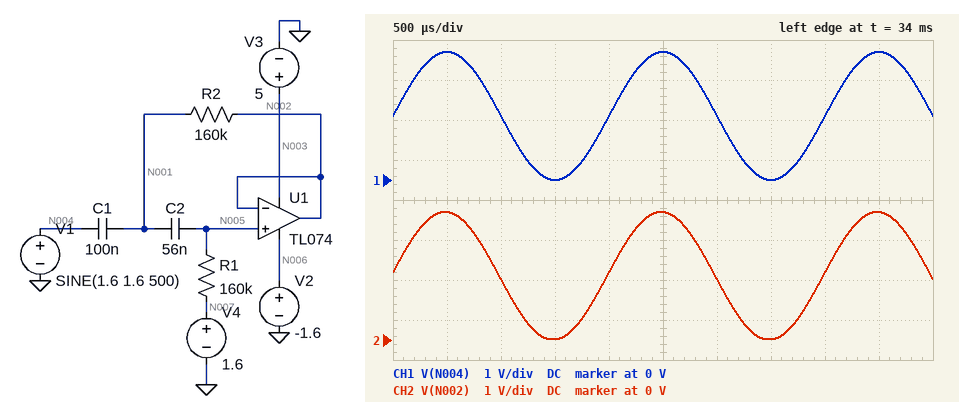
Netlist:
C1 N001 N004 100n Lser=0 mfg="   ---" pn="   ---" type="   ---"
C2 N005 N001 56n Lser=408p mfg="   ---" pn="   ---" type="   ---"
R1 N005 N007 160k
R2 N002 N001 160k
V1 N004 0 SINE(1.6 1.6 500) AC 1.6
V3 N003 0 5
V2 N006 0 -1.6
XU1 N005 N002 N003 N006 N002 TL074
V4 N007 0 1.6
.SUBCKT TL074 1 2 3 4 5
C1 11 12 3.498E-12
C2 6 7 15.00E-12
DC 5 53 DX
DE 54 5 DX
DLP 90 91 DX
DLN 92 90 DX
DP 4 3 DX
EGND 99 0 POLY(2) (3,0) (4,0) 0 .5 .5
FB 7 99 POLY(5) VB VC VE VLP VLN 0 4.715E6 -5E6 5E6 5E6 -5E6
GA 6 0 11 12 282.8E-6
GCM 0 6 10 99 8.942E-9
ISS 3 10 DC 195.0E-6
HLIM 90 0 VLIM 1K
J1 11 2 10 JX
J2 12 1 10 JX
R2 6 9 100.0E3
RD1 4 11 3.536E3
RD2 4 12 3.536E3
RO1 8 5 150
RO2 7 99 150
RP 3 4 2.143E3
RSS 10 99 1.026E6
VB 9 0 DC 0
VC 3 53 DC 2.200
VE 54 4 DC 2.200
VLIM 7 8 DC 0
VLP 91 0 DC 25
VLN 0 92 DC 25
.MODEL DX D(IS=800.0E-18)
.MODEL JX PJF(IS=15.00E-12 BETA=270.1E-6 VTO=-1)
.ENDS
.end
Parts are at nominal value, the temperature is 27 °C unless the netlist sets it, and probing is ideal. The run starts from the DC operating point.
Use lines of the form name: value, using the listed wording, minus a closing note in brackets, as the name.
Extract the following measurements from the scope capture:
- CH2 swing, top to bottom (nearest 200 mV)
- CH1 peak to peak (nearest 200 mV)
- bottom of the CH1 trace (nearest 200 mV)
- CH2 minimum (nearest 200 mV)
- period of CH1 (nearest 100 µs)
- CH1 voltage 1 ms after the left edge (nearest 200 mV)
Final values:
CH2 swing, top to bottom: 3.2 V
CH1 peak to peak: 3.2 V
bottom of the CH1 trace: 0 V
CH2 minimum: 0 V
period of CH1: 2.0 ms
CH1 voltage 1 ms after the left edge: 1.6 V
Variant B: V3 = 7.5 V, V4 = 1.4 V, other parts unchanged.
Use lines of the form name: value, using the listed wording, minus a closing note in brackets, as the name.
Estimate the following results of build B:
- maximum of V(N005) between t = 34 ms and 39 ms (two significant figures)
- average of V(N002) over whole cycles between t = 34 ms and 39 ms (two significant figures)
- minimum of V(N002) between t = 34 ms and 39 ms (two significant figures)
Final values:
maximum of V(N005) between t = 34 ms and 39 ms: 3.0 V
average of V(N002) over whole cycles between t = 34 ms and 39 ms: 1.4 V
minimum of V(N002) between t = 34 ms and 39 ms: -41 mV
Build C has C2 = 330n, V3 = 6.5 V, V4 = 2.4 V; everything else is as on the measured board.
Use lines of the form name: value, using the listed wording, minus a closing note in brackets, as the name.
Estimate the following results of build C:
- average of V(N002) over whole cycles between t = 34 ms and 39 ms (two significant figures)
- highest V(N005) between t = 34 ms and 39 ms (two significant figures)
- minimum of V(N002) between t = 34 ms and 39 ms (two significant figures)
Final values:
average of V(N002) over whole cycles between t = 34 ms and 39 ms: 2.4 V
highest V(N005) between t = 34 ms and 39 ms: 4.0 V
minimum of V(N002) between t = 34 ms and 39 ms: 800 mV
